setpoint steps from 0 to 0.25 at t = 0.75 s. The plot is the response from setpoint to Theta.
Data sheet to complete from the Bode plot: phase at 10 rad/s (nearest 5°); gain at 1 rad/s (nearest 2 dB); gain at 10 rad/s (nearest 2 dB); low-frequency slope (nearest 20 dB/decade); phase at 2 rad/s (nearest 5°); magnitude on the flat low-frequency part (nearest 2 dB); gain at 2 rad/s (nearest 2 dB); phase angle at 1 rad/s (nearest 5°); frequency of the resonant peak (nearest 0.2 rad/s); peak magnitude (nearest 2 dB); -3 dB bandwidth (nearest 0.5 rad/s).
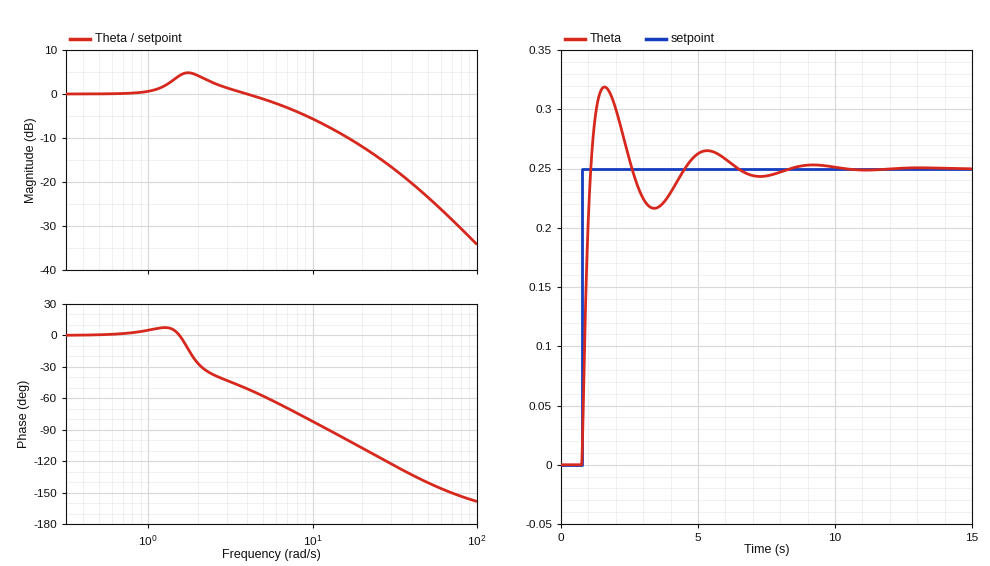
-80°
0 dB
-6 dB
0 dB/decade
-25°
0 dB
4 dB
5°
1.8 rad/s
4 dB
7.0 rad/s
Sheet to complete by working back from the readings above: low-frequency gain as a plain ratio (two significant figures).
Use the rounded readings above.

1.0
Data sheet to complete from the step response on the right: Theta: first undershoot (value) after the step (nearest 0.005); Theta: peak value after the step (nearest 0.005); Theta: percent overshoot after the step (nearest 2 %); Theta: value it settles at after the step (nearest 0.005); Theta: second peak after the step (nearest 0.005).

0.215
0.320
28 %
0.250
0.265
